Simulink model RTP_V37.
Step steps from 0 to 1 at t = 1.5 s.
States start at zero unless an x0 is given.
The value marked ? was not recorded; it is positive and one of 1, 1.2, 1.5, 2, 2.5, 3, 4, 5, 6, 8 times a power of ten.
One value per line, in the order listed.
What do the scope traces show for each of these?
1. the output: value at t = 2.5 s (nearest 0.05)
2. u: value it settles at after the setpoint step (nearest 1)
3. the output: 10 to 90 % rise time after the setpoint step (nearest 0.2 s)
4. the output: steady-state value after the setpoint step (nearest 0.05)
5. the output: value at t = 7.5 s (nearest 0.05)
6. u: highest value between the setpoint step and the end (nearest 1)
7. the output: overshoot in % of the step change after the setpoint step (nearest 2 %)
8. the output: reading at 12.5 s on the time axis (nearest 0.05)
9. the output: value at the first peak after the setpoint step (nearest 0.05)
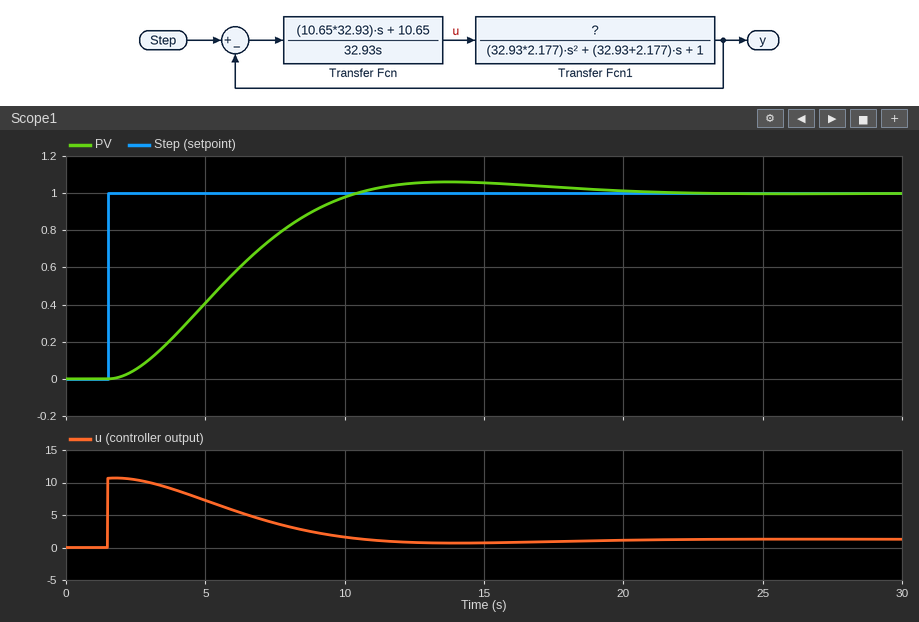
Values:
0.05
1
5.8 s
1.00
0.75
11
6 %
1.05
1.05
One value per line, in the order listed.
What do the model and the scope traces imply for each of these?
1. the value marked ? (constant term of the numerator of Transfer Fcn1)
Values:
0.8
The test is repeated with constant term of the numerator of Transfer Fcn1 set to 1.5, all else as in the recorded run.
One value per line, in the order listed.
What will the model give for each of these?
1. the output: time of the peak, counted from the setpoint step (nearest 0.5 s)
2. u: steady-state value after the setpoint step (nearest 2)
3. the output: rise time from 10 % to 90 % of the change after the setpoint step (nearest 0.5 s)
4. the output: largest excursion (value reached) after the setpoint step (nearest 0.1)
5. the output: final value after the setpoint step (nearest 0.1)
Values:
7.5 s
0
3.5 s
1.2
1.0
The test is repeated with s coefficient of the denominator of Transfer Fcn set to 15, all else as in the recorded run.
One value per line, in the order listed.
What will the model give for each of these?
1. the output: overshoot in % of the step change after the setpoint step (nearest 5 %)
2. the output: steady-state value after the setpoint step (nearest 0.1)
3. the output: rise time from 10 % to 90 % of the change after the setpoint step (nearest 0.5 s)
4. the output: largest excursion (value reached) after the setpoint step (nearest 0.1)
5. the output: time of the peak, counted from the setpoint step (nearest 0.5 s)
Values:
20 %
1.0
3.0 s
1.2
7.0 s
